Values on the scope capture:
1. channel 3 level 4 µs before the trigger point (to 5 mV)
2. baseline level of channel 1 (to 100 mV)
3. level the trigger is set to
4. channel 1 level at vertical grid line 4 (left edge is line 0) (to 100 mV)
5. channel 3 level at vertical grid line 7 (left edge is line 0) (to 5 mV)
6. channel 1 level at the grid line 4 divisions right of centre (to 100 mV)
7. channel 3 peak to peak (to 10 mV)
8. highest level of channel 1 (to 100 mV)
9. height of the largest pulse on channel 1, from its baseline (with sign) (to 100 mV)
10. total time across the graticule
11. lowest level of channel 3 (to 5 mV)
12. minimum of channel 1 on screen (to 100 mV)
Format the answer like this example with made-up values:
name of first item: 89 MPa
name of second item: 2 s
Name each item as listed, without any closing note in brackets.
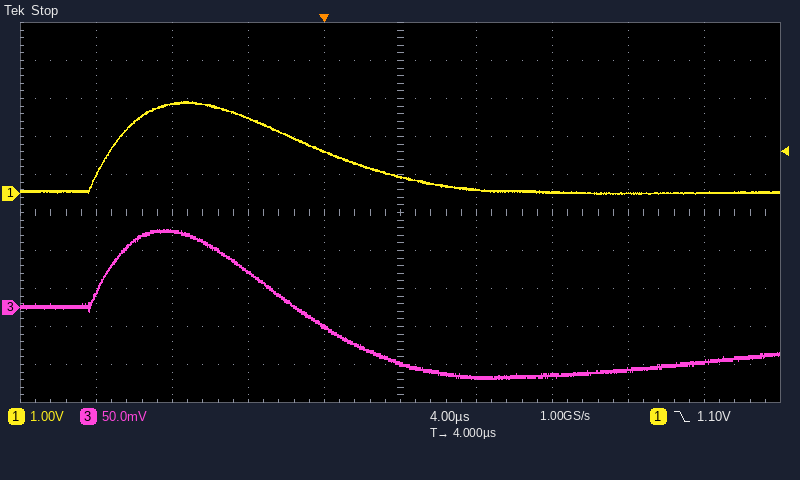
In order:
channel 3 level 4 µs before the trigger point: 45 mV
baseline level of channel 1: 0.0 V
level the trigger is set to: 1.10 V
channel 1 level at vertical grid line 4 (left edge is line 0): 1.1 V
channel 3 level at vertical grid line 7 (left edge is line 0): -90 mV
channel 1 level at the grid line 4 divisions right of centre: 0.0 V
channel 3 peak to peak: 200 mV
highest level of channel 1: 2.4 V
height of the largest pulse on channel 1, from its baseline (with sign): +2.4 V
total time across the graticule: 40 µs
lowest level of channel 3: -95 mV
minimum of channel 1 on screen: 0.0 V
